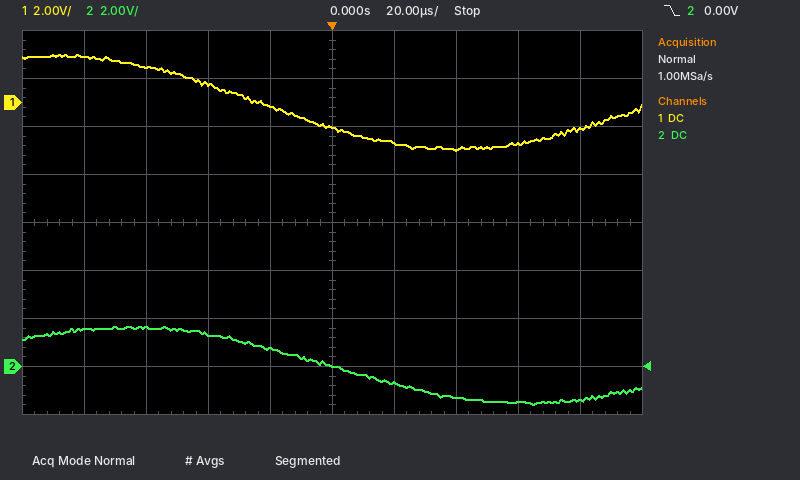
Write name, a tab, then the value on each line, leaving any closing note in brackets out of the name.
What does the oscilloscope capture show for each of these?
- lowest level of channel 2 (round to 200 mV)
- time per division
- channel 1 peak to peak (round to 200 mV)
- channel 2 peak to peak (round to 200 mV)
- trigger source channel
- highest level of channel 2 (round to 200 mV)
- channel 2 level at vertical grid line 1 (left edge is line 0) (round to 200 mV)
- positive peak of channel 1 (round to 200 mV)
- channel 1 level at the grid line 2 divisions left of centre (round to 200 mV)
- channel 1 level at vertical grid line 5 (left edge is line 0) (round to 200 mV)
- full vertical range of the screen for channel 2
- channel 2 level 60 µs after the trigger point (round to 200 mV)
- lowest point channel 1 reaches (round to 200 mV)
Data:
lowest level of channel 2	-1.6 V
time per division	20 µs
channel 1 peak to peak	4.0 V
channel 2 peak to peak	3.2 V
trigger source channel	channel 2
highest level of channel 2	1.6 V
channel 2 level at vertical grid line 1 (left edge is line 0)	1.6 V
positive peak of channel 1	2.0 V
channel 1 level at the grid line 2 divisions left of centre	800 mV
channel 1 level at vertical grid line 5 (left edge is line 0)	-1.0 V
full vertical range of the screen for channel 2	16 V
channel 2 level 60 µs after the trigger point	-1.4 V
lowest point channel 1 reaches	-2.0 V
